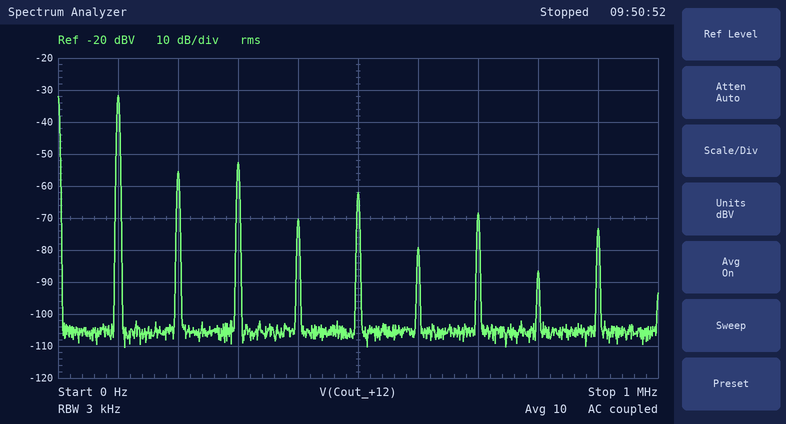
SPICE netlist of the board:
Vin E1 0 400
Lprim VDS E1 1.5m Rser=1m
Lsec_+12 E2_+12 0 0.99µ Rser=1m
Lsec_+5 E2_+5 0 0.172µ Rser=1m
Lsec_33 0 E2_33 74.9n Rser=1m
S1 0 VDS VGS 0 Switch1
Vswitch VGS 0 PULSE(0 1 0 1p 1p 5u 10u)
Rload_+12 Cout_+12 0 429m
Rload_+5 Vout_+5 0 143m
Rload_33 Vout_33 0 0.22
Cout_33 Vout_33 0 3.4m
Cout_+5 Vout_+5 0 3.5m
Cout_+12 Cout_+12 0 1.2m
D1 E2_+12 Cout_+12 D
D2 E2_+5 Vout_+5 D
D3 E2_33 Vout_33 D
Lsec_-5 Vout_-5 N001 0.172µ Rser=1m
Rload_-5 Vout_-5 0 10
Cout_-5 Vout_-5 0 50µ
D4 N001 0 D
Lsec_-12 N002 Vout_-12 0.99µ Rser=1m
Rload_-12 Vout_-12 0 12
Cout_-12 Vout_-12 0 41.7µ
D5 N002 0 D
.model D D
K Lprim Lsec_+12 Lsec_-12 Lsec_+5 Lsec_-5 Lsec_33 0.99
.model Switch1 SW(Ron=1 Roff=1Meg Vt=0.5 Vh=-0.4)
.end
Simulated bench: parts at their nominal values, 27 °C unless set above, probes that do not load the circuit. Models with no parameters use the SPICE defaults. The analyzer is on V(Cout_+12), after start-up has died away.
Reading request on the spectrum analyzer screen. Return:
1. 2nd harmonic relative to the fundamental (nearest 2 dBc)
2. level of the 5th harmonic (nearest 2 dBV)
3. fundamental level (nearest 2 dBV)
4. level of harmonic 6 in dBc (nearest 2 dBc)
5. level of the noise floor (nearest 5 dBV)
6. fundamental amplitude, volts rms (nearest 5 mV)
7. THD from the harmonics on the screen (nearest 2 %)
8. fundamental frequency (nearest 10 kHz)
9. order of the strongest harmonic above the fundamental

-24 dBc
-62 dBV
-32 dBV
-48 dBc
-105 dBV
25 mV
12 %
100 kHz
3
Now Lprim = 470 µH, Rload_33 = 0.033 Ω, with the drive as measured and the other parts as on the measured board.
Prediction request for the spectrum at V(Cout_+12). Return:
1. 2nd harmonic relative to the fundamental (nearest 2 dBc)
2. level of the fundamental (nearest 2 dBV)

-26 dBc
-26 dBV
